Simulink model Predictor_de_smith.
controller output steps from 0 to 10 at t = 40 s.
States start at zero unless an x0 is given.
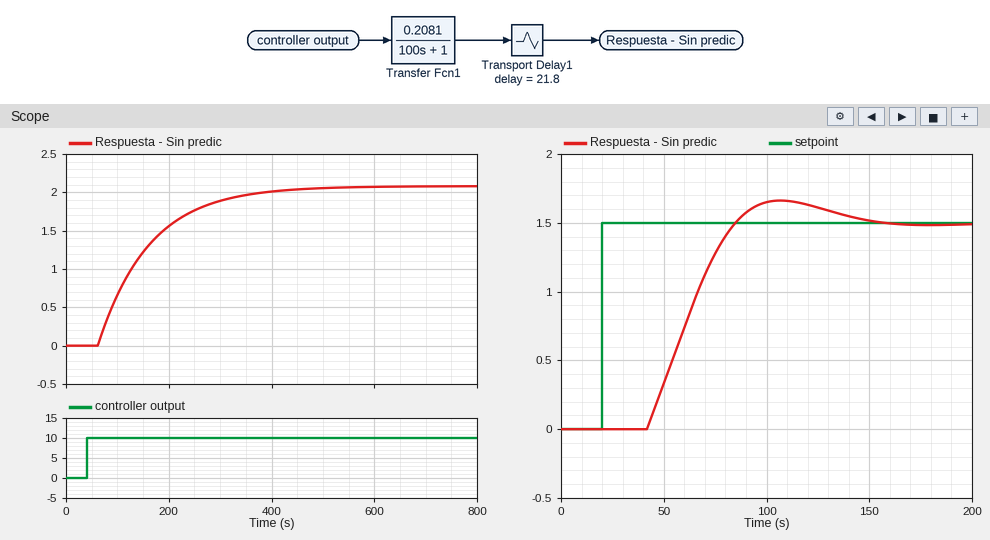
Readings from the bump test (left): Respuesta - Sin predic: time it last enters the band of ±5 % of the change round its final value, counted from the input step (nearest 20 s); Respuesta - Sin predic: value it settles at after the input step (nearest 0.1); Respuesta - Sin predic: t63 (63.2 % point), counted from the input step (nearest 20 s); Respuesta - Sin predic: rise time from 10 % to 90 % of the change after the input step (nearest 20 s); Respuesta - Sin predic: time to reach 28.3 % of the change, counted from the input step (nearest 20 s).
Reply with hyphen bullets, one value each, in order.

- 320 s
- 2.1
- 120 s
- 220 s
- 60 s
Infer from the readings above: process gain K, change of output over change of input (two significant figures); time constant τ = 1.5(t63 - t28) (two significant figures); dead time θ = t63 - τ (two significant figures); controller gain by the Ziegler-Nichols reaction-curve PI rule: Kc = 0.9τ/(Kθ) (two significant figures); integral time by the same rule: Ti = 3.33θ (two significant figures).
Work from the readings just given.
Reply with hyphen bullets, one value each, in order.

- 0.21
- 90 s
- 30 s
- 13
- 100 s
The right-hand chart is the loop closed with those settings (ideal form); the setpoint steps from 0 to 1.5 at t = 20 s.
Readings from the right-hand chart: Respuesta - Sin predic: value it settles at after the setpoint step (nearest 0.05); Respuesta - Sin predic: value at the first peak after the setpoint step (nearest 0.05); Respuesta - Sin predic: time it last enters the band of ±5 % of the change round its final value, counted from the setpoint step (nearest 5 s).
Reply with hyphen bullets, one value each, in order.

- 1.50
- 1.65
- 115 s
